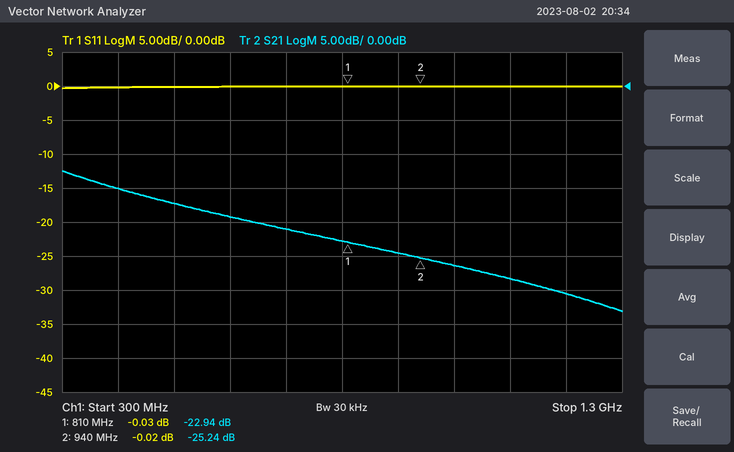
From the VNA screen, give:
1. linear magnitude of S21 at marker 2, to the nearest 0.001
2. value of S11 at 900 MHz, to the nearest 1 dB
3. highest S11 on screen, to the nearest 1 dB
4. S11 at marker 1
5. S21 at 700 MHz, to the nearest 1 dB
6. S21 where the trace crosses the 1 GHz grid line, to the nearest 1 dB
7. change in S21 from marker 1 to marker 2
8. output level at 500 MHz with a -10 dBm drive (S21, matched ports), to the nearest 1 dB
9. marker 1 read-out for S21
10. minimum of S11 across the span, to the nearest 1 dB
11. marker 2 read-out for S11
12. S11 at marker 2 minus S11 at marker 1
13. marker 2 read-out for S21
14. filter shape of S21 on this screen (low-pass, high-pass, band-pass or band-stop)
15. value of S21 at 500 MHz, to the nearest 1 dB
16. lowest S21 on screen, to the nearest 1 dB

0.055
0 dB
0 dB
-0.03 dB
-21 dB
-26 dB
-2.30 dB
-27 dBm
-22.94 dB
0 dB
-0.02 dB
0.01 dB
-25.24 dB
low-pass
-17 dB
-33 dB
